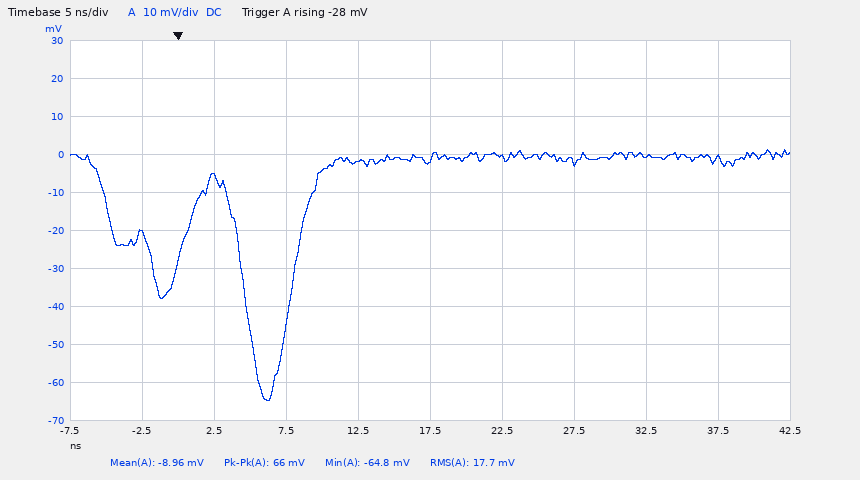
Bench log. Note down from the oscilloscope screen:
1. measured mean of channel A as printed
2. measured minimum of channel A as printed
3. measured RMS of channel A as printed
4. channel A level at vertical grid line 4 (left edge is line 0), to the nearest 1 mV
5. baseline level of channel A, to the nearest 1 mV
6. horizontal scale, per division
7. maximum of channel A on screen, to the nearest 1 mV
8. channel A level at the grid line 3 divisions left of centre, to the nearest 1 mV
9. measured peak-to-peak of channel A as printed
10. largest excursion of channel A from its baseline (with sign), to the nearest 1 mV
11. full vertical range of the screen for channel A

-8.96 mV
-64.8 mV
17.7 mV
-2 mV
-1 mV
5 ns
1 mV
-6 mV
66 mV
-64 mV
100 mV
